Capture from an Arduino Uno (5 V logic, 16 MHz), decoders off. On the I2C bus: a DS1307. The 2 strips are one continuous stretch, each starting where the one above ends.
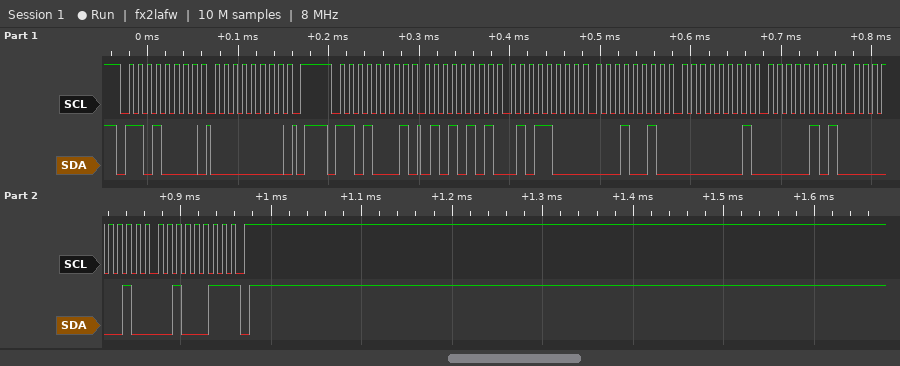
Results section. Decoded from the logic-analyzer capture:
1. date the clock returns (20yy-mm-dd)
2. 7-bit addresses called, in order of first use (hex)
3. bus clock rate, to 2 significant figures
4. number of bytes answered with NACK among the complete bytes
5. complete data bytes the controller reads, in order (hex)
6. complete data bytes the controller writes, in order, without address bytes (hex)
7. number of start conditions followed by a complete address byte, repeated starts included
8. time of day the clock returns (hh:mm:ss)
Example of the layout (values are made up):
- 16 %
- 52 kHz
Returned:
- 2023-02-05
- 0x68
- 100 kHz
- 1
- 55 58 12 01 05 02 23
- 00
- 2
- 12:58:55
